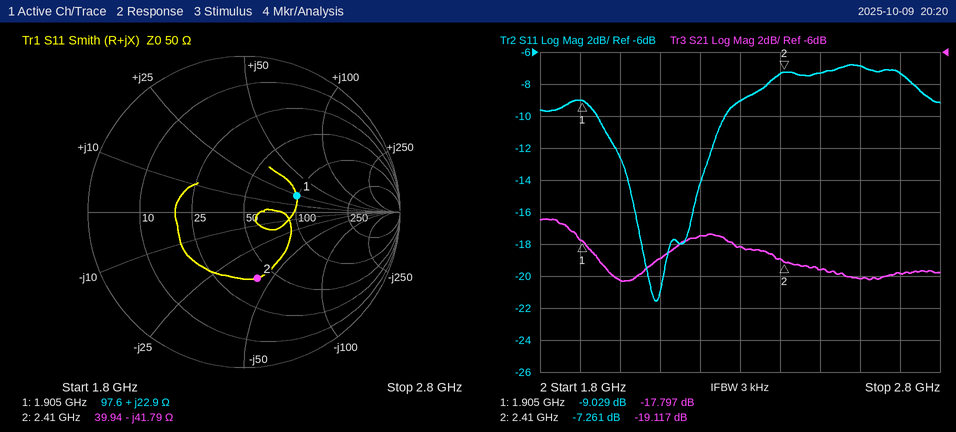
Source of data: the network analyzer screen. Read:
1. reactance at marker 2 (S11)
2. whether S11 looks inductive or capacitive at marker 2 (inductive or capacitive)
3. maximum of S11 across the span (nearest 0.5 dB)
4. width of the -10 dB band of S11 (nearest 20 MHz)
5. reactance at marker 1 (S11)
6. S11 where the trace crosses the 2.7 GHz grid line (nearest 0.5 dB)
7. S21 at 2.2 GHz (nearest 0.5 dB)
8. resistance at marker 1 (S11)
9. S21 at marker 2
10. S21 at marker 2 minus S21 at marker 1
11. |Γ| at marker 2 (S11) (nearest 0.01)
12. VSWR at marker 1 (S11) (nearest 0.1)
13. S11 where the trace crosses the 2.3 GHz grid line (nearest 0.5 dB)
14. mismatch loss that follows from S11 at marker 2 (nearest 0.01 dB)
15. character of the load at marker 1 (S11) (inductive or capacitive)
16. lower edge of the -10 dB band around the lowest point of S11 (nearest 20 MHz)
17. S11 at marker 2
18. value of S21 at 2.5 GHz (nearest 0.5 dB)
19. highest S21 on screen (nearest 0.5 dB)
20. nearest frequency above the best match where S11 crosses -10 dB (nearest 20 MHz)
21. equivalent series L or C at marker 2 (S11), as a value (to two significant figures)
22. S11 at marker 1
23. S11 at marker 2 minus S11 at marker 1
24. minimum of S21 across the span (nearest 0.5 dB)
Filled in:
-41.79 Ω
capacitive
-7.0 dB
320 MHz
+22.9 Ω
-7.5 dB
-17.5 dB
97.6 Ω
-19.117 dB
-1.320 dB
0.43
2.1
-9.0 dB
0.90 dB
inductive
1.94 GHz
-7.261 dB
-19.5 dB
-16.5 dB
2.26 GHz
1.6 pF
-9.029 dB
1.768 dB
-20.5 dB
